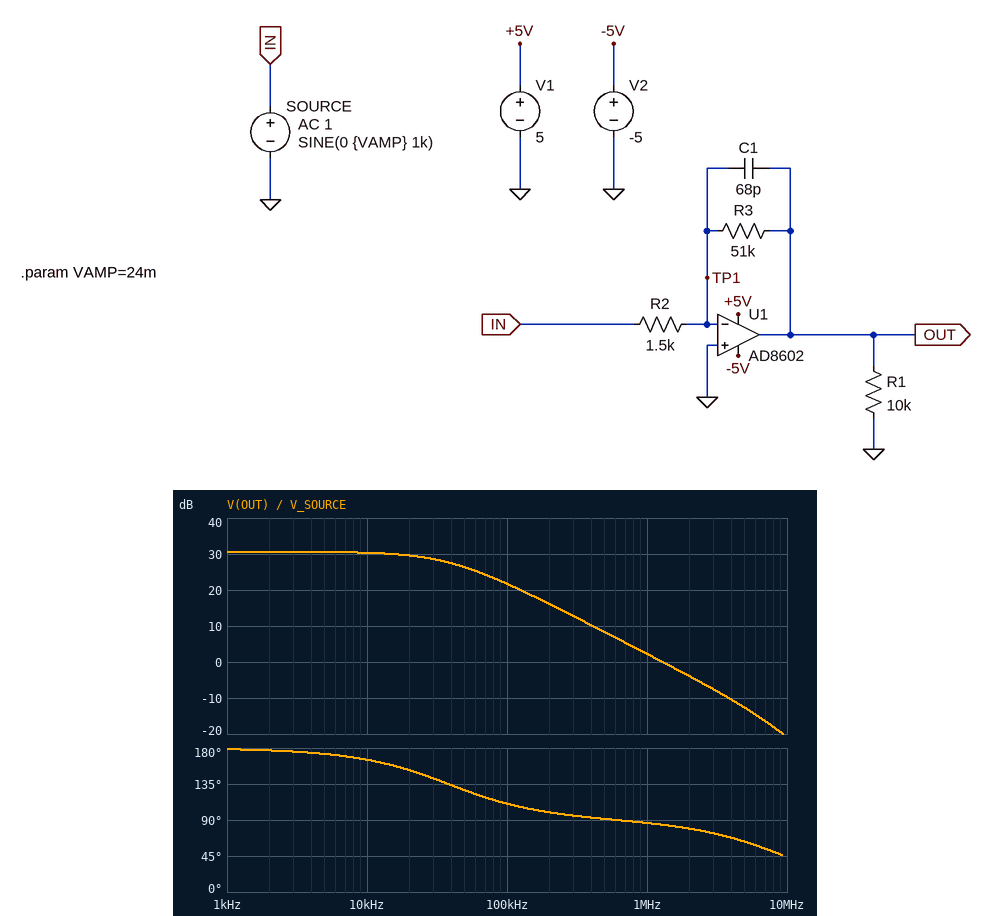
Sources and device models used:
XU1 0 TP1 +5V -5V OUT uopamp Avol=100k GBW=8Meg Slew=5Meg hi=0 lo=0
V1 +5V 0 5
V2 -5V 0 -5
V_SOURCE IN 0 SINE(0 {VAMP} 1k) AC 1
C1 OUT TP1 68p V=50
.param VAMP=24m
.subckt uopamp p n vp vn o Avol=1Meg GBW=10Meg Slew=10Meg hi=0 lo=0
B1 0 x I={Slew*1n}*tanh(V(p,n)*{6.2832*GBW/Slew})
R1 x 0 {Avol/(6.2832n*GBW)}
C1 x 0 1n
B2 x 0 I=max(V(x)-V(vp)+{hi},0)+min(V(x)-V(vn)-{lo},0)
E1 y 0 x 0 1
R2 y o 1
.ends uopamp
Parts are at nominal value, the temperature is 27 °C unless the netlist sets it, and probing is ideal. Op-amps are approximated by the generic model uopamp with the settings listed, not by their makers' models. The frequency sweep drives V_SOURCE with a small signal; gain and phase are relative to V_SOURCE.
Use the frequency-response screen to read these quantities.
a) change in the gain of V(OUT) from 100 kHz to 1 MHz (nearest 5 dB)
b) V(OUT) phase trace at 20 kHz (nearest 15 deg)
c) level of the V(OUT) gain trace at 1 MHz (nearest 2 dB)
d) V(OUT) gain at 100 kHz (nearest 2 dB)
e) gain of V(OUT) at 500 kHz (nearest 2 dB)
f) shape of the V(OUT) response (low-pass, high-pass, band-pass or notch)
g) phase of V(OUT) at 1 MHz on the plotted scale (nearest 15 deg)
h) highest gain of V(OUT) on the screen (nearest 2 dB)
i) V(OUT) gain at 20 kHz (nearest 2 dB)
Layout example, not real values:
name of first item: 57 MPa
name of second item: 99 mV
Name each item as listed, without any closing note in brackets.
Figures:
change in the gain of V(OUT) from 100 kHz to 1 MHz: -20 dB
V(OUT) phase trace at 20 kHz: 150 deg
level of the V(OUT) gain trace at 1 MHz: 2 dB
V(OUT) gain at 100 kHz: 22 dB
gain of V(OUT) at 500 kHz: 8 dB
shape of the V(OUT) response: low-pass
phase of V(OUT) at 1 MHz on the plotted scale: 90 deg
highest gain of V(OUT) on the screen: 30 dB
V(OUT) gain at 20 kHz: 30 dB
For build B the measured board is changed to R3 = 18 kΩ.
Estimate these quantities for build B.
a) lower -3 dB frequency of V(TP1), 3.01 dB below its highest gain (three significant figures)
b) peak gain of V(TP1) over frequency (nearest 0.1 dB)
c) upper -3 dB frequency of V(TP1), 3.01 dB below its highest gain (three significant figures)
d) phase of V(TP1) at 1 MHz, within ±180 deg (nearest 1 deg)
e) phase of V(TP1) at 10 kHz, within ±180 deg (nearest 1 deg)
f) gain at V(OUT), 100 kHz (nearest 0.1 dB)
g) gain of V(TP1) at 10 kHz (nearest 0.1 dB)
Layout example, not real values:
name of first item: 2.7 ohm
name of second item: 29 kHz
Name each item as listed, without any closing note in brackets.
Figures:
lower -3 dB frequency of V(TP1), 3.01 dB below its highest gain: 106 kHz
peak gain of V(TP1) over frequency: -15.9 dB
upper -3 dB frequency of V(TP1), 3.01 dB below its highest gain: 9.79 MHz
phase of V(TP1) at 1 MHz, within ±180 deg: 0 deg
phase of V(TP1) at 10 kHz, within ±180 deg: 84 deg
gain at V(OUT), 100 kHz: 18.9 dB
gain of V(TP1) at 10 kHz: -36.5 dB
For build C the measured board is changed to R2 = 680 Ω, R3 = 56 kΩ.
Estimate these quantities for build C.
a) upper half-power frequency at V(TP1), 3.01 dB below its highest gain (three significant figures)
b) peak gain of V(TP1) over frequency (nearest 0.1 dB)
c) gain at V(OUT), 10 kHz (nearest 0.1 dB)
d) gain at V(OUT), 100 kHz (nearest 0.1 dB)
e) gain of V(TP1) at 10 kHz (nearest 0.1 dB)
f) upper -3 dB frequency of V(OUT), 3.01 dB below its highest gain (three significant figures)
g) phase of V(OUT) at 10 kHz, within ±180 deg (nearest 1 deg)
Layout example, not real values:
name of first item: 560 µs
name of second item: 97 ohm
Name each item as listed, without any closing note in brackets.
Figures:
upper half-power frequency at V(TP1), 3.01 dB below its highest gain: 11.5 MHz
peak gain of V(TP1) over frequency: -10.5 dB
gain at V(OUT), 10 kHz: 37.8 dB
gain at V(OUT), 100 kHz: 27.3 dB
gain of V(TP1) at 10 kHz: -20.2 dB
upper -3 dB frequency of V(OUT), 3.01 dB below its highest gain: 29.2 kHz
phase of V(OUT) at 10 kHz, within ±180 deg: 161 deg
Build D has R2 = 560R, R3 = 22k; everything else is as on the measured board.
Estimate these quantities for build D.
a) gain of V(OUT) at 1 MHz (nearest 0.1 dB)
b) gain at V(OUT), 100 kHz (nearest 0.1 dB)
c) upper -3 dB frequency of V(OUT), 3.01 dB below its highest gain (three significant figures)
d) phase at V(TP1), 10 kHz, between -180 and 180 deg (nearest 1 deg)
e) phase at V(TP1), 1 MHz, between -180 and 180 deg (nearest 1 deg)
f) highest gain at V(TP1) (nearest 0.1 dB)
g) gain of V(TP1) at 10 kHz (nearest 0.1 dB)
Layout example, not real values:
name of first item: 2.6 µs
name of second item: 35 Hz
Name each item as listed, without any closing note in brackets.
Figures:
gain of V(OUT) at 1 MHz: 8.7 dB
gain at V(OUT), 100 kHz: 27.0 dB
upper -3 dB frequency of V(OUT), 3.01 dB below its highest gain: 69.7 kHz
phase at V(TP1), 10 kHz, between -180 and 180 deg: 81 deg
phase at V(TP1), 1 MHz, between -180 and 180 deg: -1 deg
highest gain at V(TP1): -9.4 dB
gain of V(TP1) at 10 kHz: -26.3 dB
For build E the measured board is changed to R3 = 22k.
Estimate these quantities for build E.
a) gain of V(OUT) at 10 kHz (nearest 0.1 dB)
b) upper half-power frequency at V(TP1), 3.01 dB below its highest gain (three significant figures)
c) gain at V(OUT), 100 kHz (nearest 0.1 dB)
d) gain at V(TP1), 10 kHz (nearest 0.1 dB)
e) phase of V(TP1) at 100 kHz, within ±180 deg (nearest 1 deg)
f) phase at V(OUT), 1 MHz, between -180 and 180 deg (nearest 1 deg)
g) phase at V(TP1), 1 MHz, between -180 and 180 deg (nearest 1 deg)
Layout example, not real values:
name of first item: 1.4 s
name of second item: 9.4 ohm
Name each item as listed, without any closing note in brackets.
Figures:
gain of V(OUT) at 10 kHz: 23.3 dB
upper half-power frequency at V(TP1), 3.01 dB below its highest gain: 9.75 MHz
gain at V(OUT), 100 kHz: 19.8 dB
gain at V(TP1), 10 kHz: -34.8 dB
phase of V(TP1) at 100 kHz, within ±180 deg: 41 deg
phase at V(OUT), 1 MHz, between -180 and 180 deg: 89 deg
phase at V(TP1), 1 MHz, between -180 and 180 deg: -1 deg
